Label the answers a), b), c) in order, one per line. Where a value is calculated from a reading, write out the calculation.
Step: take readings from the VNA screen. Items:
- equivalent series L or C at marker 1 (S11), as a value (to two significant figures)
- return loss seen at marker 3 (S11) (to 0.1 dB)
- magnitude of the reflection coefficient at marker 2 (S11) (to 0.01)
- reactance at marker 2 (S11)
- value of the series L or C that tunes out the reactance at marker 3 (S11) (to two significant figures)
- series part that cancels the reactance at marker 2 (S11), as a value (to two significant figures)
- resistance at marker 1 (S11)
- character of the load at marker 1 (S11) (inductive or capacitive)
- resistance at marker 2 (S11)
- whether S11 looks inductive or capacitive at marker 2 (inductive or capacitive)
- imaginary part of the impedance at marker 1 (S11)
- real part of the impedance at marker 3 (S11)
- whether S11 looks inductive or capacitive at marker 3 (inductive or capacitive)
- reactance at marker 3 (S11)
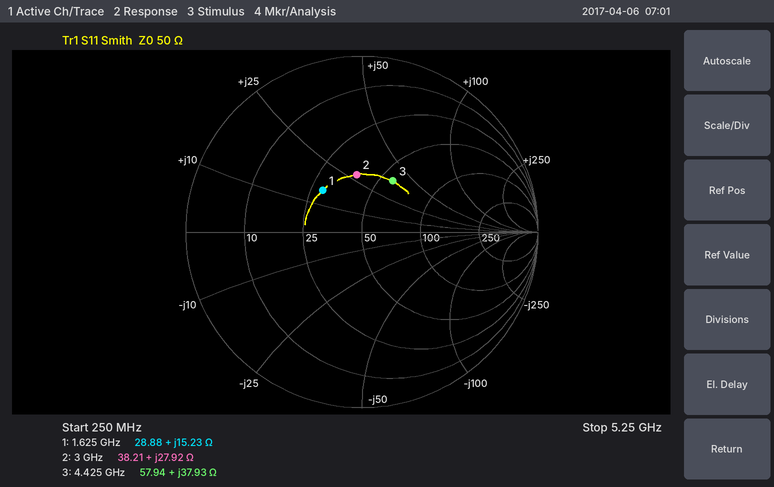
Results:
a) L = 15.23 Ω/(2π × 1.625 GHz) ≈ 1.5 nH
b) 9.4 dB
c) 0.33
d) +27.92 Ω
e) C = 1/(2π × 4.425 GHz × 37.93 Ω) ≈ 948 fF, so 950 fF to two significant figures
f) C = 1/(2π × 3 GHz × 27.92 Ω) ≈ 1.9 pF
g) 28.88 Ω
h) inductive
i) 38.21 Ω
j) inductive
k) +15.23 Ω
l) 57.94 Ω
m) inductive
n) +37.93 Ω
